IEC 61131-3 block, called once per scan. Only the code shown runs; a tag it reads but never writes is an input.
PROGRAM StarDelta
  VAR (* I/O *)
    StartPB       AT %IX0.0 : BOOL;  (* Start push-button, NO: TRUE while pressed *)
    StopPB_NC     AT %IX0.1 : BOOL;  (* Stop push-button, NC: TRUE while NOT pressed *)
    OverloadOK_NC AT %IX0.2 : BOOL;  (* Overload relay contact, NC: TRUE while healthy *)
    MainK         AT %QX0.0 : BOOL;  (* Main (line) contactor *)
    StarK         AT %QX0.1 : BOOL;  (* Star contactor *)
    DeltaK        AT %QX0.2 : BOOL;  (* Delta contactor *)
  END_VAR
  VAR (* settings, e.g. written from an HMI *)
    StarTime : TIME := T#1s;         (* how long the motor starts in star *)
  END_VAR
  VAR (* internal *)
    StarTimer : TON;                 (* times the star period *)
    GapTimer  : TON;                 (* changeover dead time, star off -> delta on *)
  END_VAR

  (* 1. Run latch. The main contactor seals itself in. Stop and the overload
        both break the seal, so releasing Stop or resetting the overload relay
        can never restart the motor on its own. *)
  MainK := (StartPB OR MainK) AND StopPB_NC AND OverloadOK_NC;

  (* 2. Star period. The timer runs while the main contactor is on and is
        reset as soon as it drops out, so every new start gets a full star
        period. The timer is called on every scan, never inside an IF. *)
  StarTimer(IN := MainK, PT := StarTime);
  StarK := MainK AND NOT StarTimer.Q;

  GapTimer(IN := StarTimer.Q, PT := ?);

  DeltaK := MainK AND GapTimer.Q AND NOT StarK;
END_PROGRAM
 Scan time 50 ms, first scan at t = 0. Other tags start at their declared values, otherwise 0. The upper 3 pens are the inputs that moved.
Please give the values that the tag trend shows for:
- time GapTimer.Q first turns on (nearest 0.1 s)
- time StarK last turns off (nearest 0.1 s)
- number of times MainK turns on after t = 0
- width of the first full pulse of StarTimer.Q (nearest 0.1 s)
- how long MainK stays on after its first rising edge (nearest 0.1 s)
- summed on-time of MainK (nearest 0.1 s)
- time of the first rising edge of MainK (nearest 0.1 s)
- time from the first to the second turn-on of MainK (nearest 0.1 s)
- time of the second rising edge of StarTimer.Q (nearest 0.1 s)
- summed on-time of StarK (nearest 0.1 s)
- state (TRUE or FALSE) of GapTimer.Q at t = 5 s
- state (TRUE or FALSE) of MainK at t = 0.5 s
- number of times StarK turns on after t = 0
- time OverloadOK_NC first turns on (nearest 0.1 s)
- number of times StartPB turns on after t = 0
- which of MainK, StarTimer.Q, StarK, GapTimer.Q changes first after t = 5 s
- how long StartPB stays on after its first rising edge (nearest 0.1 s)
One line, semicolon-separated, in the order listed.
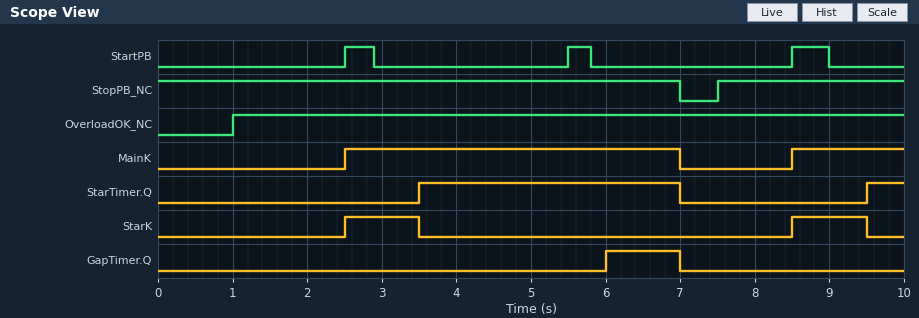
6.0 s; 9.5 s; 2; 3.5 s; 4.5 s; 6.0 s; 2.5 s; 6.0 s; 9.5 s; 2.0 s; FALSE; FALSE; 2; 1.0 s; 3; GapTimer.Q; 0.4 s
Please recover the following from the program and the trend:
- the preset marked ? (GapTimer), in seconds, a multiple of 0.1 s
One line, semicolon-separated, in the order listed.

2.5 s
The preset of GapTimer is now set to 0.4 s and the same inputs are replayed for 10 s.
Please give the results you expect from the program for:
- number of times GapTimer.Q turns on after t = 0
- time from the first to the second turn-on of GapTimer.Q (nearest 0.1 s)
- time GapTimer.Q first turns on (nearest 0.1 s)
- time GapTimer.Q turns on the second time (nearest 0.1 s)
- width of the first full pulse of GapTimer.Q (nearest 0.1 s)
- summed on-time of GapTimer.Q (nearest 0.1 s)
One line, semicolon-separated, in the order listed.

2; 6.0 s; 3.9 s; 9.9 s; 3.1 s; 3.2 s
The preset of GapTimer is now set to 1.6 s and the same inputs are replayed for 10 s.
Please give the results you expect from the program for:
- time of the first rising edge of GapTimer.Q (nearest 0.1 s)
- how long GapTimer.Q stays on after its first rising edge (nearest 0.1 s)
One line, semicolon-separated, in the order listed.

5.1 s; 1.9 s
